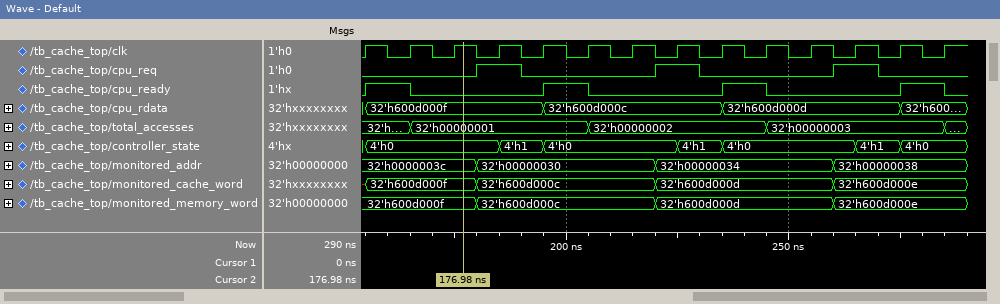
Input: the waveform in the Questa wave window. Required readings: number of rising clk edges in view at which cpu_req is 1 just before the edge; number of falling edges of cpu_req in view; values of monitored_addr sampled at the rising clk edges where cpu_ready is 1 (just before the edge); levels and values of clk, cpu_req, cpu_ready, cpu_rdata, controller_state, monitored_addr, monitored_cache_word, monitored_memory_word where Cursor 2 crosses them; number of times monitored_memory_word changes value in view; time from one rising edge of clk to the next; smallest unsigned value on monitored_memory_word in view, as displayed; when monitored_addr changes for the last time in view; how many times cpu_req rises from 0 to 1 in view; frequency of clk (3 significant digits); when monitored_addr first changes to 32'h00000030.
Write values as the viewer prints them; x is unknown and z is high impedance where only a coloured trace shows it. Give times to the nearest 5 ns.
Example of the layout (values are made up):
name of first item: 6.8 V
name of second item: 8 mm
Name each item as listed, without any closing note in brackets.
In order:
number of rising clk edges in view at which cpu_req is 1 just before the edge: 3
number of falling edges of cpu_req in view: 3
values of monitored_addr sampled at the rising clk edges where cpu_ready is 1: 32'h0000003c, 32'h00000030, 32'h00000034, 32'h00000038
levels and values of clk, cpu_req, cpu_ready, cpu_rdata, controller_state, monitored_addr, monitored_cache_word, monitored_memory_word where Cursor 2 crosses them: clk=1, cpu_req=0, cpu_ready=0, cpu_rdata=32'h600d000f, controller_state=4'h0, monitored_addr=32'h0000003c, monitored_cache_word=32'h600d000f, monitored_memory_word=32'h600d000f
number of times monitored_memory_word changes value in view: 3
time from one rising edge of clk to the next: 10 ns
smallest unsigned value on monitored_memory_word in view, as displayed: 32'h600d000c
when monitored_addr changes for the last time in view: 260 ns
how many times cpu_req rises from 0 to 1 in view: 3
frequency of clk: 100 MHz
when monitored_addr first changes to 32'h00000030: 180 ns
